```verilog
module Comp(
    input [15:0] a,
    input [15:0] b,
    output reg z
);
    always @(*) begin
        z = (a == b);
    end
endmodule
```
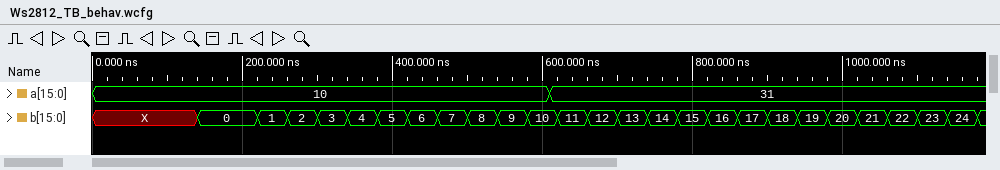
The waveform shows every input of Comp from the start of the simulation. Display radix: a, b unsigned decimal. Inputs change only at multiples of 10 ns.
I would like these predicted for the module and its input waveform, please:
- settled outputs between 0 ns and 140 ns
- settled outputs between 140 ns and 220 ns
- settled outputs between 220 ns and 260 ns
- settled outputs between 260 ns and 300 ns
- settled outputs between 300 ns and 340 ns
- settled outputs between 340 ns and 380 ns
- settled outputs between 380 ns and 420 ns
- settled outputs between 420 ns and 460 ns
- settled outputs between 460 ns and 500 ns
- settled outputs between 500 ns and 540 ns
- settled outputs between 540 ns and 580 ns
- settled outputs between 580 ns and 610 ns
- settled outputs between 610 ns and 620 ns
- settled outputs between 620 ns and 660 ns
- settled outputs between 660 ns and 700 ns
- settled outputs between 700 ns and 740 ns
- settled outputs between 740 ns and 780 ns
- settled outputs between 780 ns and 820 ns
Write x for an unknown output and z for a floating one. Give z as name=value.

z=x
z=0
z=0
z=0
z=0
z=0
z=0
z=0
z=0
z=0
z=0
z=1
z=0
z=0
z=0
z=0
z=0
z=0
